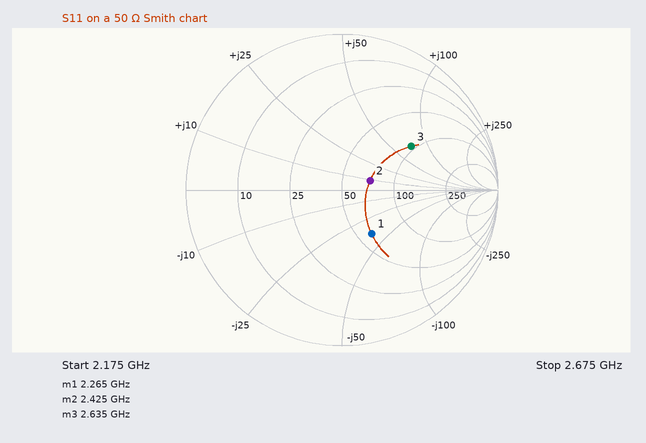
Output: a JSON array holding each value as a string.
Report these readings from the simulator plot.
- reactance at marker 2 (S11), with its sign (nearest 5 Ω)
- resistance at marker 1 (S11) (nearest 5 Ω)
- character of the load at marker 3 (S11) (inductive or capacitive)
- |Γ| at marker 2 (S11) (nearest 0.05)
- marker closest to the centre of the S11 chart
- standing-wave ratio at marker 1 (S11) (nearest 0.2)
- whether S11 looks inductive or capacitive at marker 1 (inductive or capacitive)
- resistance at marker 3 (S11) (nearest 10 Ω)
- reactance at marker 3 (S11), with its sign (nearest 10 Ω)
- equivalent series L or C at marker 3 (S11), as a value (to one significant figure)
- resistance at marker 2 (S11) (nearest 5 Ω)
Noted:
["+10 Ω", "60 Ω", "inductive", "0.20", "marker 2", "2.0", "capacitive", "90 Ω", "+70 Ω", "4 nH", "70 Ω"]
